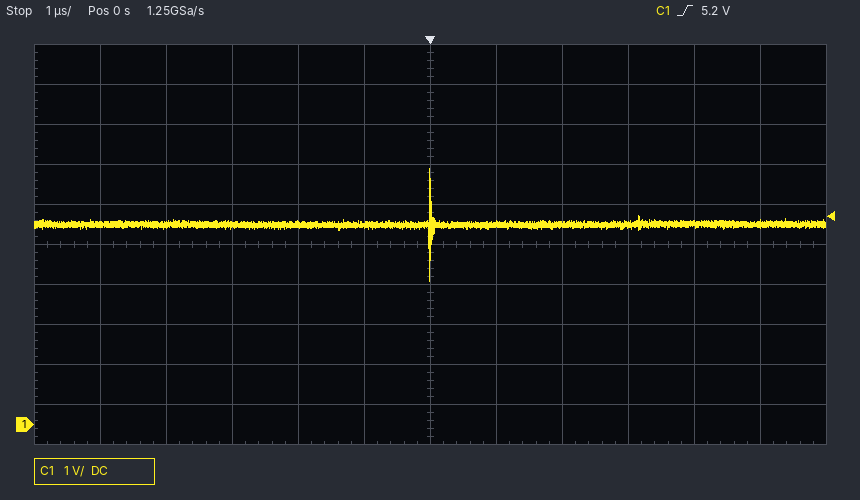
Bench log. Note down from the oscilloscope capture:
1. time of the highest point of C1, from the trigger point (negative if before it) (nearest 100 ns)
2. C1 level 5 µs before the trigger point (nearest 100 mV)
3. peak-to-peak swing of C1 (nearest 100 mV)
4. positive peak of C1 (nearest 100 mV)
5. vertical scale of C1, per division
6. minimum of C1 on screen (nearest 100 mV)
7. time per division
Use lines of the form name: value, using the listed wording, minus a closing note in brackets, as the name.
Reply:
time of the highest point of C1, from the trigger point (negative if before it): 0.0 µs
C1 level 5 µs before the trigger point: 5.0 V
peak-to-peak swing of C1: 2.8 V
positive peak of C1: 6.4 V
vertical scale of C1, per division: 1 V
minimum of C1 on screen: 3.6 V
time per division: 1 µs
